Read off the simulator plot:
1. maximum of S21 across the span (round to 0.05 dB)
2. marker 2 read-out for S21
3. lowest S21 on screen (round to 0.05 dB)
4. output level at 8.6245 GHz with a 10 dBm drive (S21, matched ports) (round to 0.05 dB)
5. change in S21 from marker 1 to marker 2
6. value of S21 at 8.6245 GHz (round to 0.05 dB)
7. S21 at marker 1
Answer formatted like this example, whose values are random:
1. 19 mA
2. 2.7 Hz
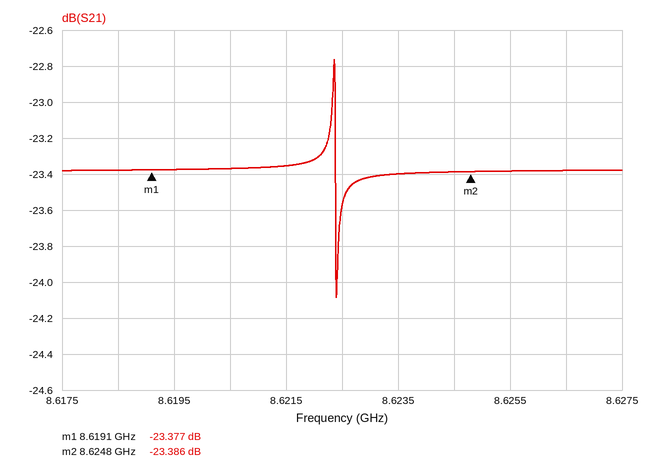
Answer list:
1. -22.75 dB
2. -23.386 dB
3. -24.10 dB
4. -13.40 dBm
5. -0.009 dB
6. -23.40 dB
7. -23.377 dB
